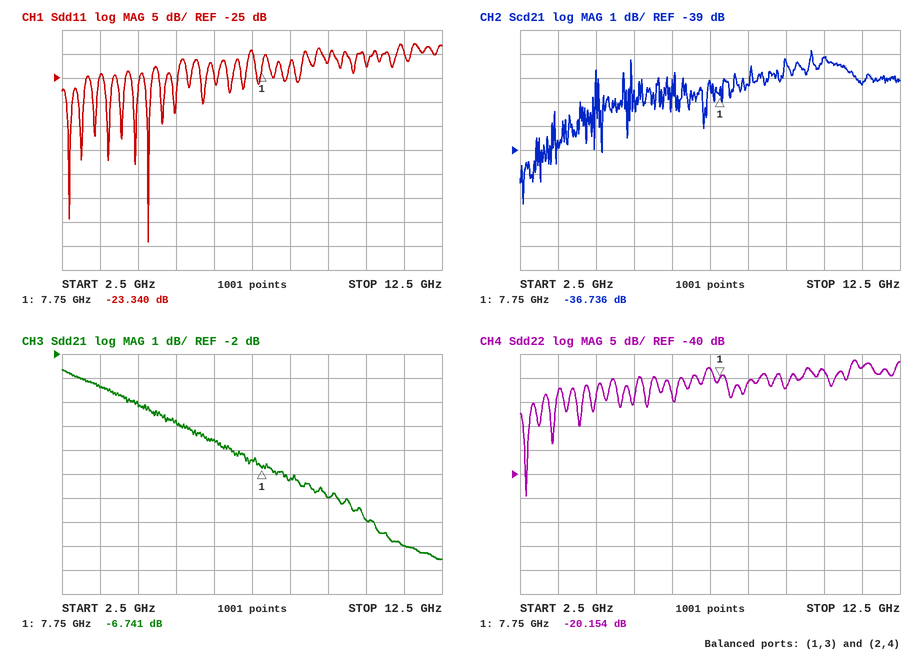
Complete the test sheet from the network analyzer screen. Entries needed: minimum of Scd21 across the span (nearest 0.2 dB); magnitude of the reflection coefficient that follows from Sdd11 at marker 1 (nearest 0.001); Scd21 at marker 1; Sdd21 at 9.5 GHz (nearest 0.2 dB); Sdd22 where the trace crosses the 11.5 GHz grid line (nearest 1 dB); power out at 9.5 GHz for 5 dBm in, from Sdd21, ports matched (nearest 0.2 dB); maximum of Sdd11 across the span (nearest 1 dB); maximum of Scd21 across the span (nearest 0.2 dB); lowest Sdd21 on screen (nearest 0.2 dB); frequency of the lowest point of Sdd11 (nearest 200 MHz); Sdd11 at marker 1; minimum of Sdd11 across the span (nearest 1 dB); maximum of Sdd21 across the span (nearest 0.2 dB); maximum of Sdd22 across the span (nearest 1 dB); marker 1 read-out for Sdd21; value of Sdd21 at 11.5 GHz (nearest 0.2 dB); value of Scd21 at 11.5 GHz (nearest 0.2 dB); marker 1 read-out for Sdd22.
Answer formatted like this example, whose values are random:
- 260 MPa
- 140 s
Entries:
- -41.2 dB
- 0.068
- -36.736 dB
- -8.0 dB
- -18 dB
- -3.0 dBm
- -18 dB
- -34.8 dB
- -10.6 dB
- 4.8 GHz
- -23.340 dB
- -59 dB
- -2.6 dB
- -16 dB
- -6.741 dB
- -10.0 dB
- -36.2 dB
- -20.154 dB
